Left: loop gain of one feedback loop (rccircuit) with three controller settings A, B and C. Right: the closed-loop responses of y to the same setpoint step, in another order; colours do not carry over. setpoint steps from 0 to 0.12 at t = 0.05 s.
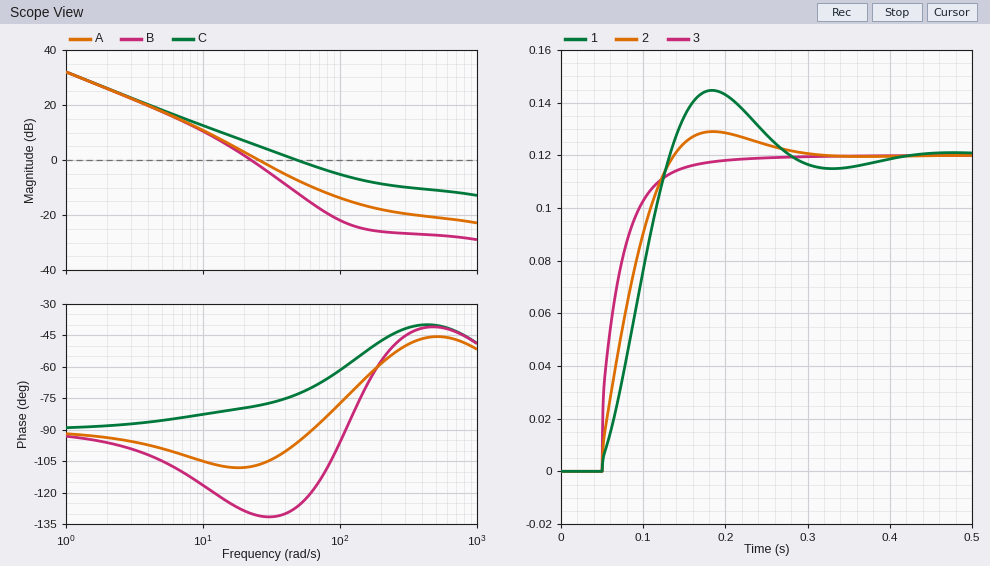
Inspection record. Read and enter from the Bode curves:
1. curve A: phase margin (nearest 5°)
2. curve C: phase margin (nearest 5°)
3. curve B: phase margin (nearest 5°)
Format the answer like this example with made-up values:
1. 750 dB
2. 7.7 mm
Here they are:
1. 75°
2. 105°
3. 50°
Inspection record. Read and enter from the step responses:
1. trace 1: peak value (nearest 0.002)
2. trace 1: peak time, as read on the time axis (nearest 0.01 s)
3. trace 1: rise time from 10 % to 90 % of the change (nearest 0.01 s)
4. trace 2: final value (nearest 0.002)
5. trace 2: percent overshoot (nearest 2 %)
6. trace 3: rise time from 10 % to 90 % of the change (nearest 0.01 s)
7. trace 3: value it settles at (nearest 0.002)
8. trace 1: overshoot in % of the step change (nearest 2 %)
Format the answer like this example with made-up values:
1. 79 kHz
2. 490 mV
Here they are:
1. 0.144
2. 0.18 s
3. 0.06 s
4. 0.120
5. 8 %
6. 0.06 s
7. 0.120
8. 20 %
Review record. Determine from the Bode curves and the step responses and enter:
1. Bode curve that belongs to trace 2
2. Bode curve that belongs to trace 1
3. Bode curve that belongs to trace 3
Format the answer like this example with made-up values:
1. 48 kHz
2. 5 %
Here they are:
1. A
2. B
3. C
